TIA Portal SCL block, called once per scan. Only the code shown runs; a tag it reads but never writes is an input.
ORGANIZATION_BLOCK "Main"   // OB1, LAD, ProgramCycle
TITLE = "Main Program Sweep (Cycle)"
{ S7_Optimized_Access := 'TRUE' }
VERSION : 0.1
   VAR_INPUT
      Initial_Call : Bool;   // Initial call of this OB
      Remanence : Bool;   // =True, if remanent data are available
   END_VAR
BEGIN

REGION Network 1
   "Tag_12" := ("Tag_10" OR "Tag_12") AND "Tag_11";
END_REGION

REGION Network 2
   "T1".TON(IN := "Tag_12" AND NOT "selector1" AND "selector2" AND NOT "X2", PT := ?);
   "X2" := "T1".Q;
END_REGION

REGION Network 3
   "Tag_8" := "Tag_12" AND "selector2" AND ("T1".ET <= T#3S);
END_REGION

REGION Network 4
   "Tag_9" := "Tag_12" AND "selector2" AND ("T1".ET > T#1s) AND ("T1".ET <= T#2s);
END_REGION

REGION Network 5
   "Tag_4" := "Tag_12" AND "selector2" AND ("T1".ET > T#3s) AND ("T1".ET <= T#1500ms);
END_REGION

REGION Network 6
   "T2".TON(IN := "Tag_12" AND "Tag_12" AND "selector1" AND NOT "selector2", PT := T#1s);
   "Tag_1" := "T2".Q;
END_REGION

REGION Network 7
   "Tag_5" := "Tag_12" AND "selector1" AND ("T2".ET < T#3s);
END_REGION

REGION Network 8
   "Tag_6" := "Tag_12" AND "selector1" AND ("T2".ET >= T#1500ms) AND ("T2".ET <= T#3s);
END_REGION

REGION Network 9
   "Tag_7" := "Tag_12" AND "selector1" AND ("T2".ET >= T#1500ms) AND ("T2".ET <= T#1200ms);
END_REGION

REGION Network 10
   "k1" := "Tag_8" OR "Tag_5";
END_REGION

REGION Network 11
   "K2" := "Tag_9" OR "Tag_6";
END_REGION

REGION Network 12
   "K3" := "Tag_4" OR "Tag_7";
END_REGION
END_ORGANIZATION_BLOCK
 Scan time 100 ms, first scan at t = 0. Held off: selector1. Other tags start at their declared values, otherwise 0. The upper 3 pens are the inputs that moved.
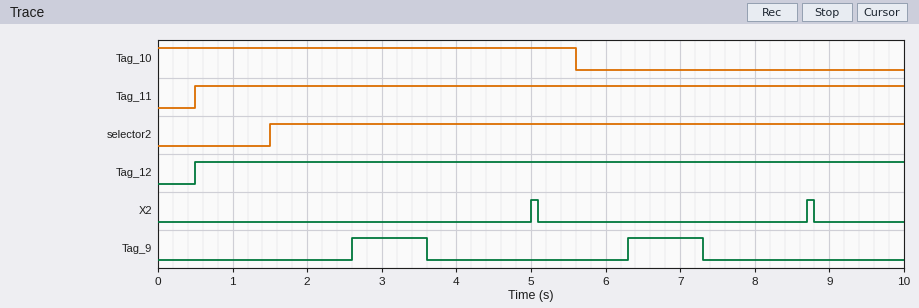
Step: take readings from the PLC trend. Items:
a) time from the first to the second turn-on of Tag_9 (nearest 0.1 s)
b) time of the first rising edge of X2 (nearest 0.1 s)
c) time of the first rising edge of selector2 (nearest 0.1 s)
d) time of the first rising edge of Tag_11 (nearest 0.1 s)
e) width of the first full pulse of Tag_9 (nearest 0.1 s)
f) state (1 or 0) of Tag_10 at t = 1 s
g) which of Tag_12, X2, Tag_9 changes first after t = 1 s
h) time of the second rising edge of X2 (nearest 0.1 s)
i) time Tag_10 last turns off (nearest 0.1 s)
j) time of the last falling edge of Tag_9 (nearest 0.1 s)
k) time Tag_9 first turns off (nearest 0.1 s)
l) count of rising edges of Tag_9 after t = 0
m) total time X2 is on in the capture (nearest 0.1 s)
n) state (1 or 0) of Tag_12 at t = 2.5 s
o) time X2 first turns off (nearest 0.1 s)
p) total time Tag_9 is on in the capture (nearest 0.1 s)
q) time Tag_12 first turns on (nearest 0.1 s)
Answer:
3.7 s
5.0 s
1.5 s
0.5 s
1.0 s
1
Tag_9
8.7 s
5.6 s
7.3 s
3.6 s
2
0.2 s
1
5.1 s
2.0 s
0.5 s
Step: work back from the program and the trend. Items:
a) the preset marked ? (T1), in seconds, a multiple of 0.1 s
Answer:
3.5 s
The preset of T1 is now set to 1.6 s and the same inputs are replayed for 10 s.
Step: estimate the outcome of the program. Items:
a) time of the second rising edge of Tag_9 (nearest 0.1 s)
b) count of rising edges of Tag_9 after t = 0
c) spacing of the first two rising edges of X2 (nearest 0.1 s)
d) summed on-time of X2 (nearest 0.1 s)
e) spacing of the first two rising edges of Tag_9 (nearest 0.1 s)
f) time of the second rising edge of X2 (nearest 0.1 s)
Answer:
4.4 s
5
1.8 s
0.4 s
1.8 s
4.9 s
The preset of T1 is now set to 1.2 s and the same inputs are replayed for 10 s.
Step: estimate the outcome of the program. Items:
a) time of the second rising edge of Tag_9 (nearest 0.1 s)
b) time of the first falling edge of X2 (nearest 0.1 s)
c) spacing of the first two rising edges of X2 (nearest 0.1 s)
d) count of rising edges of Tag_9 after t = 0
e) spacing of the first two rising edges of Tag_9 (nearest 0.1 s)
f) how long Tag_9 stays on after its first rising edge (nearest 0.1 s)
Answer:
4.0 s
2.8 s
1.4 s
6
1.4 s
0.2 s
